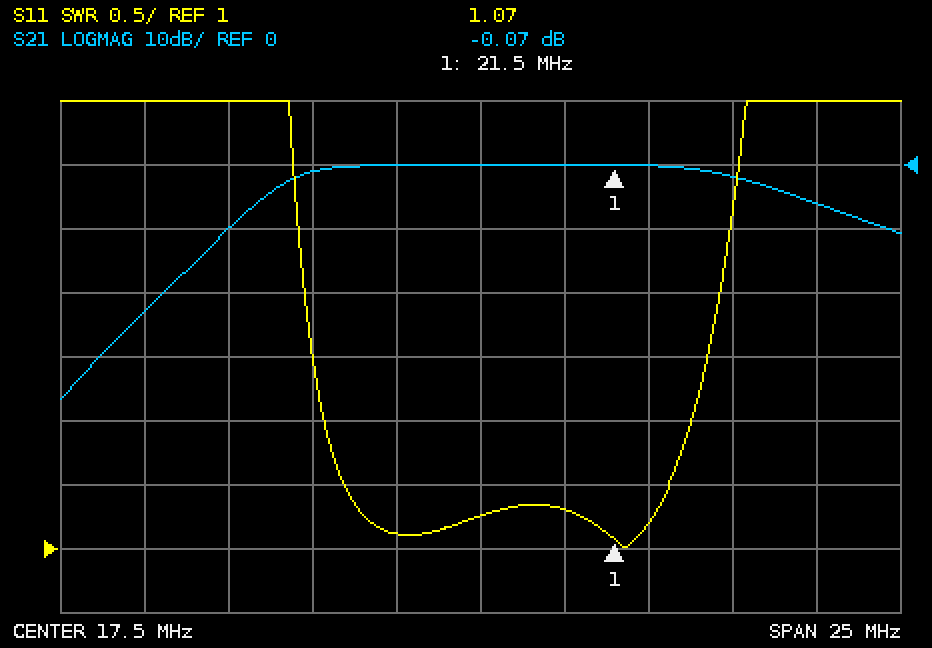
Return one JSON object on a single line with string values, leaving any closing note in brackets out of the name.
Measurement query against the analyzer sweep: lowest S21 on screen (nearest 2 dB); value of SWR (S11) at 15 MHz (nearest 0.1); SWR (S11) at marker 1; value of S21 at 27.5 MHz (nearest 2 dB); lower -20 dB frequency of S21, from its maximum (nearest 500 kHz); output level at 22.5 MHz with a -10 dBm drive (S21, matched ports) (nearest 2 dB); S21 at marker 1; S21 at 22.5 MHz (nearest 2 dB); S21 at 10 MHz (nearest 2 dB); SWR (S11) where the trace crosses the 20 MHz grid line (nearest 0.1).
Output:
{"lowest S21 on screen": "-36 dB", "value of SWR (S11) at 15 MHz": "1.1", "SWR (S11) at marker 1": "1.07", "value of S21 at 27.5 MHz": "-6 dB", "lower -20 dB frequency of S21, from its maximum": "8.0 MHz", "output level at 22.5 MHz with a -10 dBm drive (S21, matched ports)": "-10 dBm", "S21 at marker 1": "-0.07 dB", "S21 at 22.5 MHz": "0 dB", "S21 at 10 MHz": "-10 dB", "SWR (S11) where the trace crosses the 20 MHz grid line": "1.3"}
